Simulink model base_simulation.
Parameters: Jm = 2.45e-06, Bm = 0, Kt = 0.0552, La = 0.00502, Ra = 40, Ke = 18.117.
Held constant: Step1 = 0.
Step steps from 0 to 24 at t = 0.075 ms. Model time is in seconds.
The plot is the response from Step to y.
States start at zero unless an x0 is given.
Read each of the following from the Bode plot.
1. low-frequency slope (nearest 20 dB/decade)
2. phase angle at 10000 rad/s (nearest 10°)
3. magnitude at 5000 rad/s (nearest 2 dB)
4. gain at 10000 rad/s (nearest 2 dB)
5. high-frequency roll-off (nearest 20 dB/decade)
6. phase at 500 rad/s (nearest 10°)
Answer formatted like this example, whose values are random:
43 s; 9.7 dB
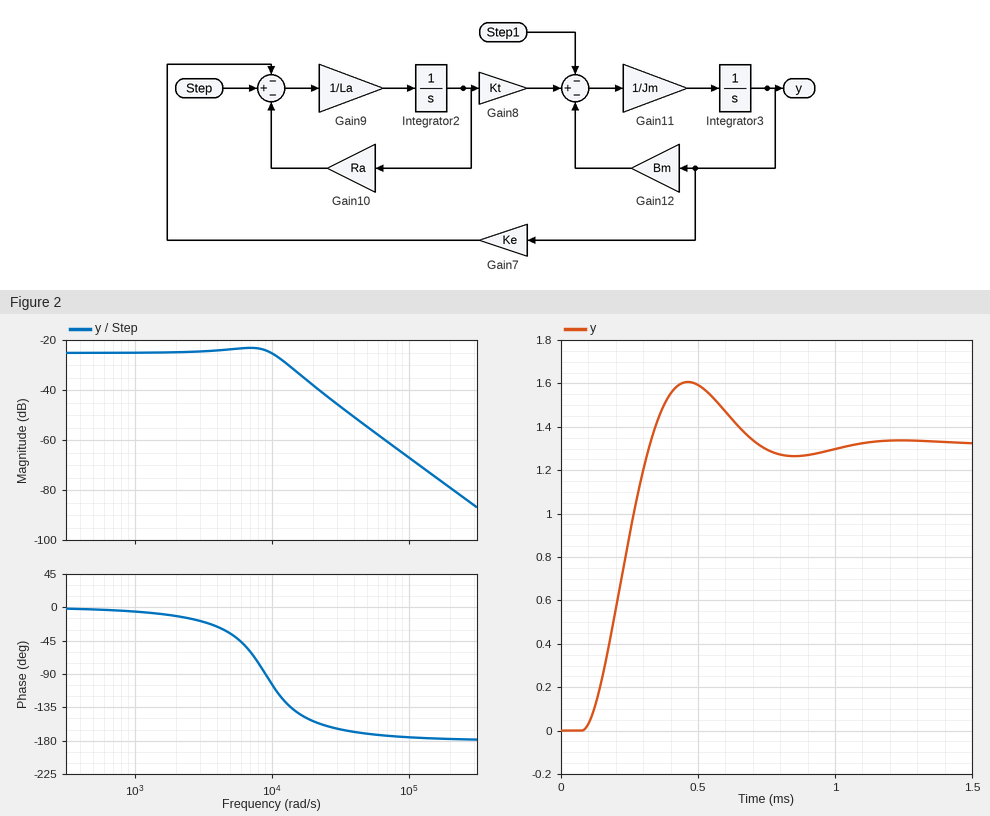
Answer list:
0 dB/decade; -100°; -24 dB; -26 dB; -40 dB/decade; 0°
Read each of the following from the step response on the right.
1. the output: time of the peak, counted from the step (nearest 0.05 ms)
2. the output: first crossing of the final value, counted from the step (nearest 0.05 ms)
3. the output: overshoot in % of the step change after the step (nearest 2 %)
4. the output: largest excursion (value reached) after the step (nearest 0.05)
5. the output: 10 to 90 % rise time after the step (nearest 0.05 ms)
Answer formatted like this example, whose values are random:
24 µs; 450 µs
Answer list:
0.40 ms; 0.25 ms; 22 %; 1.60; 0.15 ms
